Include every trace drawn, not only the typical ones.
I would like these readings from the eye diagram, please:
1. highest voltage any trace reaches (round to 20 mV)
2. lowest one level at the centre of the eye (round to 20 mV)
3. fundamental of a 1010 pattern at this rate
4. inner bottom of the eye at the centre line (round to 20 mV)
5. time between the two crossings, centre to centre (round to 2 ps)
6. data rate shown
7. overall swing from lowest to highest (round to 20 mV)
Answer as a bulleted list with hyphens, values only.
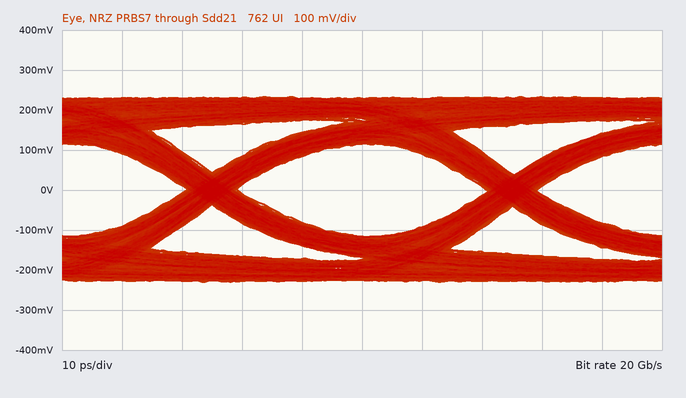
- 240 mV
- 120 mV
- 10 GHz
- -120 mV
- 50 ps
- 20 Gb/s
- 460 mV
